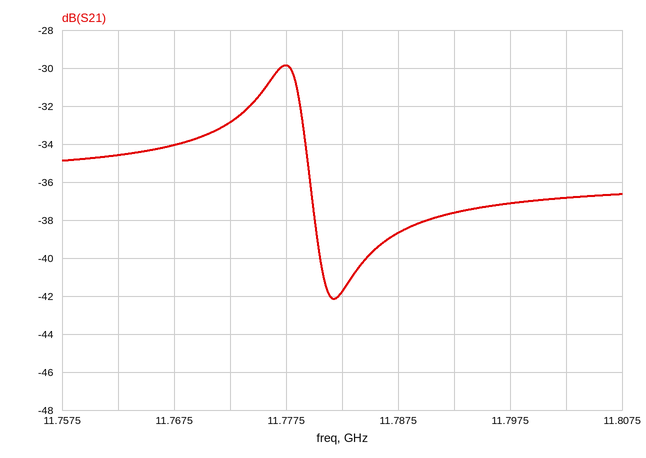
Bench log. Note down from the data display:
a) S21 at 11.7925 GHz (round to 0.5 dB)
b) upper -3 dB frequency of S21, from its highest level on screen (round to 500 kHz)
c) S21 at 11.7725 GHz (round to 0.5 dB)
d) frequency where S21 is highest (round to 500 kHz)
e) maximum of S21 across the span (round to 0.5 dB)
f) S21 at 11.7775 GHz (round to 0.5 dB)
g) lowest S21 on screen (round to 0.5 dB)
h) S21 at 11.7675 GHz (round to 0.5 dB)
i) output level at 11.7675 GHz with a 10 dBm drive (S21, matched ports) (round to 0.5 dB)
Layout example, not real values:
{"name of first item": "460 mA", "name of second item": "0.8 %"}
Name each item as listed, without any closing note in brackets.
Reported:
{"S21 at 11.7925 GHz": "-37.5 dB", "upper -3 dB frequency of S21, from its highest level on screen": "11.7790 GHz", "S21 at 11.7725 GHz": "-33.0 dB", "frequency where S21 is highest": "11.7775 GHz", "maximum of S21 across the span": "-30.0 dB", "S21 at 11.7775 GHz": "-30.0 dB", "lowest S21 on screen": "-42.0 dB", "S21 at 11.7675 GHz": "-34.0 dB", "output level at 11.7675 GHz with a 10 dBm drive (S21, matched ports)": "-24.0 dBm"}
